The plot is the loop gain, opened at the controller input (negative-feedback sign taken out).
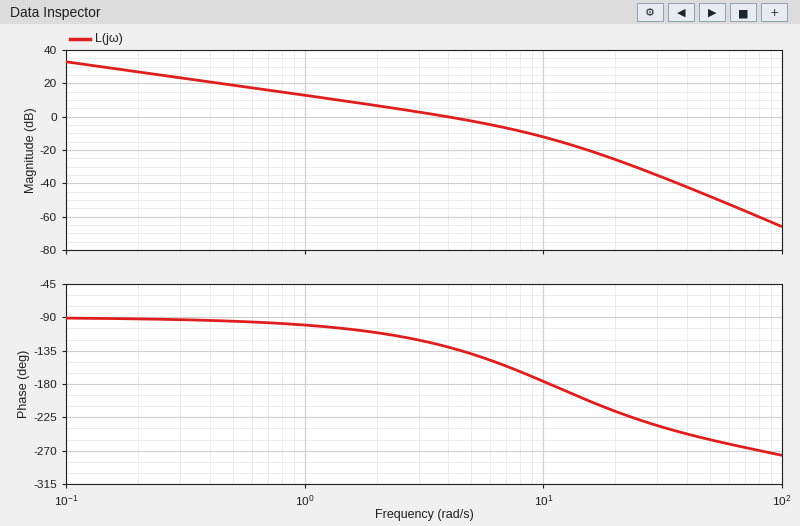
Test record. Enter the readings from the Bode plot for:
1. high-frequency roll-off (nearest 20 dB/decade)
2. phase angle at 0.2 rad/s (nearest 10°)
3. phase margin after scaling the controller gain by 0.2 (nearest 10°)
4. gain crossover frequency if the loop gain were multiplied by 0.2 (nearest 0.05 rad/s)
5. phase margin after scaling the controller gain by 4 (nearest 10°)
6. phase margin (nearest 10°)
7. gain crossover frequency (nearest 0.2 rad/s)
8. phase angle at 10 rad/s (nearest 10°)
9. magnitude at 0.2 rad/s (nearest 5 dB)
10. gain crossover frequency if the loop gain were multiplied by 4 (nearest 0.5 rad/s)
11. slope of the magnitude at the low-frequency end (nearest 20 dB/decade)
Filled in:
-60 dB/decade
-90°
80°
0.90 rad/s
0°
50°
4.0 rad/s
-180°
25 dB
10.0 rad/s
-20 dB/decade
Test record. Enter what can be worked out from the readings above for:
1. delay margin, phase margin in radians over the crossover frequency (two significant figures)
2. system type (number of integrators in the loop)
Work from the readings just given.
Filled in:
0.22 s
1
